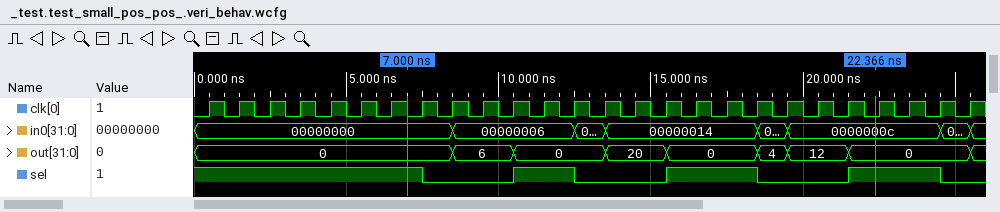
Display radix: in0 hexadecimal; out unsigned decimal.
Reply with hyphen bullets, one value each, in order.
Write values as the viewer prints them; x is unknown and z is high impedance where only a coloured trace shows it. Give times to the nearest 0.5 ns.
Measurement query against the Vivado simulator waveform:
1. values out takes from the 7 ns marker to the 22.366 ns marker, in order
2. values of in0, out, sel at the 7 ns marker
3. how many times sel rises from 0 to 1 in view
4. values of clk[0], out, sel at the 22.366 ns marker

- 0, 6, 0, 20, 0, 4, 12, 0
- in0=00000000, out=0, sel=1
- 3
- clk[0]=0, out=0, sel=1
